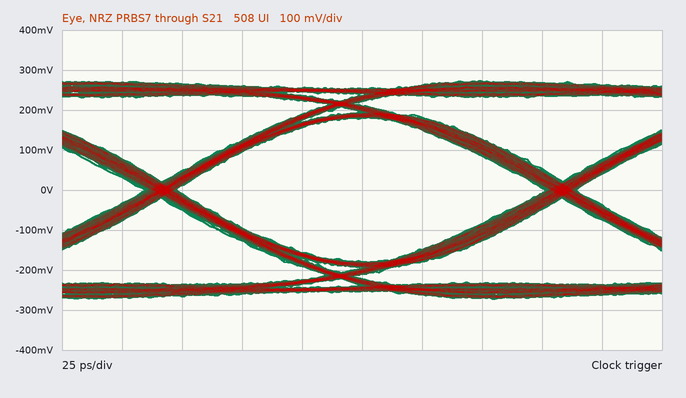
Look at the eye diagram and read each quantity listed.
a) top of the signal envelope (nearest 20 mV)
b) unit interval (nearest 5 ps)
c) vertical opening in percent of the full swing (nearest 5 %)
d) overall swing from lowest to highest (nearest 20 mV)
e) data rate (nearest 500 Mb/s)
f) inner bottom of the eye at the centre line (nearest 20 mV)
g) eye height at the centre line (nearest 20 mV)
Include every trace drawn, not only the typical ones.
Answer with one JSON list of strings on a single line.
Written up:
["280 mV", "165 ps", "65 %", "540 mV", "6.0 Gb/s", "-180 mV", "360 mV"]
